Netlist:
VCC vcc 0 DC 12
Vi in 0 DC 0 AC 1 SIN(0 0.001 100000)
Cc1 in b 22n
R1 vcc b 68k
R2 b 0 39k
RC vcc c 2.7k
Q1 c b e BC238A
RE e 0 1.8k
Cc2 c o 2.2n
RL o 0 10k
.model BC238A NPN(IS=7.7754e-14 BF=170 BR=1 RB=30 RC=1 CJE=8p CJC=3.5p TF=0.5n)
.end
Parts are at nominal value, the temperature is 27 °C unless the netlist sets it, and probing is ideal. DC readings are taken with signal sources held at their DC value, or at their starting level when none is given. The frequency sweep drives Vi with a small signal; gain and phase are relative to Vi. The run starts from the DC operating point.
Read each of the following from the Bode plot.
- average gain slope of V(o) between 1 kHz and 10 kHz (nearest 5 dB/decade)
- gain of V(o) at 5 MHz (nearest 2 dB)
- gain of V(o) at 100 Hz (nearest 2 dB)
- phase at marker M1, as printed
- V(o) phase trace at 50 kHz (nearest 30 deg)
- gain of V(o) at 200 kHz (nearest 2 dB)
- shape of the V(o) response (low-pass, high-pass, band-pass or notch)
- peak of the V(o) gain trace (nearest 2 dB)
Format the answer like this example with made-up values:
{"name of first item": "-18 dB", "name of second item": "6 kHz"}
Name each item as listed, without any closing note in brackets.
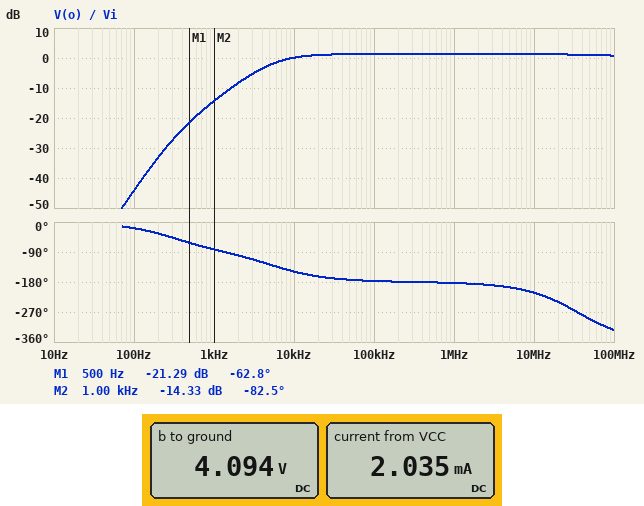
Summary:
{"average gain slope of V(o) between 1 kHz and 10 kHz": "15 dB/decade", "gain of V(o) at 5 MHz": "2 dB", "gain of V(o) at 100 Hz": "-44 dB", "phase at marker M1, as printed": "-62.8 deg", "V(o) phase trace at 50 kHz": "-180 deg", "gain of V(o) at 200 kHz": "2 dB", "shape of the V(o) response": "high-pass", "peak of the V(o) gain trace": "2 dB"}
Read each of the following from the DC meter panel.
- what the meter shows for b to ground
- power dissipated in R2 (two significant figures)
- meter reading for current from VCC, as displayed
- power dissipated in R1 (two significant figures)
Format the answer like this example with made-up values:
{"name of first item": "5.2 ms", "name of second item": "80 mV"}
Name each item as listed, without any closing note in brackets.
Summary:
{"what the meter shows for b to ground": "4.094 V", "power dissipated in R2": "430 µW", "meter reading for current from VCC, as displayed": "2.035 mA", "power dissipated in R1": "920 µW"}
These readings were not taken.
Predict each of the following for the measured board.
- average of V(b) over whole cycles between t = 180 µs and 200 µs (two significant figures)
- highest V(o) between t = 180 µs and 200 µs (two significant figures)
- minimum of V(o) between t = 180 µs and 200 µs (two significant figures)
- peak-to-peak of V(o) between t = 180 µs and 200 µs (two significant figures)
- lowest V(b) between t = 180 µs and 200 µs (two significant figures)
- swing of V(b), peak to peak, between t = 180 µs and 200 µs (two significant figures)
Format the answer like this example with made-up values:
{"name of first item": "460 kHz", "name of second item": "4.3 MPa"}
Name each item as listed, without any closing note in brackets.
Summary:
{"average of V(b) over whole cycles between t = 180 µs and 200 µs": "4.1 V", "highest V(o) between t = 180 µs and 200 µs": "1.2 mV", "minimum of V(o) between t = 180 µs and 200 µs": "-1.2 mV", "peak-to-peak of V(o) between t = 180 µs and 200 µs": "2.3 mV", "lowest V(b) between t = 180 µs and 200 µs": "4.1 V", "swing of V(b), peak to peak, between t = 180 µs and 200 µs": "2.0 mV"}
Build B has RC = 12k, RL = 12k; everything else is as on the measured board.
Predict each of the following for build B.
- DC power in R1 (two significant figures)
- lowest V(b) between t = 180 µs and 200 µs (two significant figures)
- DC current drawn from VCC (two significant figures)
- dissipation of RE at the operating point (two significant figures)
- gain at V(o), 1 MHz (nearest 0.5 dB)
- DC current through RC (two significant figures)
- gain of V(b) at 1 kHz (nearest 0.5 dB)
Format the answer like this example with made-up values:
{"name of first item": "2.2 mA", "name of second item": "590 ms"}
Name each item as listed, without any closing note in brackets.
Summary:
{"DC power in R1": "1.4 mW", "lowest V(b) between t = 180 µs and 200 µs": "2.3 V", "DC current drawn from VCC": "1.0 mA", "dissipation of RE at the operating point": "1.6 mW", "gain at V(o), 1 MHz": "-2.5 dB", "DC current through RC": "850 µA", "gain of V(b) at 1 kHz": "-13.5 dB"}
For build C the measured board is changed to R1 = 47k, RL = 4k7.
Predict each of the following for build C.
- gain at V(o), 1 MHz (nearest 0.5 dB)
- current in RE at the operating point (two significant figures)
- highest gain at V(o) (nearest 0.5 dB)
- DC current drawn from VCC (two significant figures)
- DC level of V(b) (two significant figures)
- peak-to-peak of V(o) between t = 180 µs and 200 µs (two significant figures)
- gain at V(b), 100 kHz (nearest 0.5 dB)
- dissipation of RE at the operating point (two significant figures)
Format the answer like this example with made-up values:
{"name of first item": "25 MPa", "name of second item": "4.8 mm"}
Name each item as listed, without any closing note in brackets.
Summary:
{"gain at V(o), 1 MHz": "-0.5 dB", "current in RE at the operating point": "2.5 mA", "highest gain at V(o)": "0.5 dB", "DC current drawn from VCC": "2.6 mA", "DC level of V(b)": "5.1 V", "peak-to-peak of V(o) between t = 180 µs and 200 µs": "1.9 mV", "gain at V(b), 100 kHz": "0 dB", "dissipation of RE at the operating point": "11 mW"}
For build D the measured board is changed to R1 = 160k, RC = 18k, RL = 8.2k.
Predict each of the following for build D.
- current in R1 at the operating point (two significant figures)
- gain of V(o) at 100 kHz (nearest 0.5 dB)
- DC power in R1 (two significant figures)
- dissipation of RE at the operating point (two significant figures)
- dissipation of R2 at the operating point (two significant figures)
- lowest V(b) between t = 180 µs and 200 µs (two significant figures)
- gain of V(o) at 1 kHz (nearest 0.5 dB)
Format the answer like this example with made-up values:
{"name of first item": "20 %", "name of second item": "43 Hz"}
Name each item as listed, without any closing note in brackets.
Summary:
{"current in R1 at the operating point": "64 µA", "gain of V(o) at 100 kHz": "-16.5 dB", "DC power in R1": "660 µW", "dissipation of RE at the operating point": "690 µW", "dissipation of R2 at the operating point": "75 µW", "lowest V(b) between t = 180 µs and 200 µs": "1.7 V", "gain of V(o) at 1 kHz": "-46.5 dB"}
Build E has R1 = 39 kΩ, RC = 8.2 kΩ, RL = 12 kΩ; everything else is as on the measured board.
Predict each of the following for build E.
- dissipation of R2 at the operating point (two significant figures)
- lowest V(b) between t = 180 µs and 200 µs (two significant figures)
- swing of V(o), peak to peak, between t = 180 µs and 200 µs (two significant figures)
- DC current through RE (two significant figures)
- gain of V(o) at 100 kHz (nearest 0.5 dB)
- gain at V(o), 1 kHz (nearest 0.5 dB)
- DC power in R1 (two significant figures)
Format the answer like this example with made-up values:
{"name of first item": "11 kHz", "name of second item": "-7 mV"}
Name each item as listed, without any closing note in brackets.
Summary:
{"dissipation of R2 at the operating point": "230 µW", "lowest V(b) between t = 180 µs and 200 µs": "3.0 V", "swing of V(o), peak to peak, between t = 180 µs and 200 µs": "1.7 mV", "DC current through RE": "1.3 mA", "gain of V(o) at 100 kHz": "-1.5 dB", "gain at V(o), 1 kHz": "-31.0 dB", "DC power in R1": "2.1 mW"}
